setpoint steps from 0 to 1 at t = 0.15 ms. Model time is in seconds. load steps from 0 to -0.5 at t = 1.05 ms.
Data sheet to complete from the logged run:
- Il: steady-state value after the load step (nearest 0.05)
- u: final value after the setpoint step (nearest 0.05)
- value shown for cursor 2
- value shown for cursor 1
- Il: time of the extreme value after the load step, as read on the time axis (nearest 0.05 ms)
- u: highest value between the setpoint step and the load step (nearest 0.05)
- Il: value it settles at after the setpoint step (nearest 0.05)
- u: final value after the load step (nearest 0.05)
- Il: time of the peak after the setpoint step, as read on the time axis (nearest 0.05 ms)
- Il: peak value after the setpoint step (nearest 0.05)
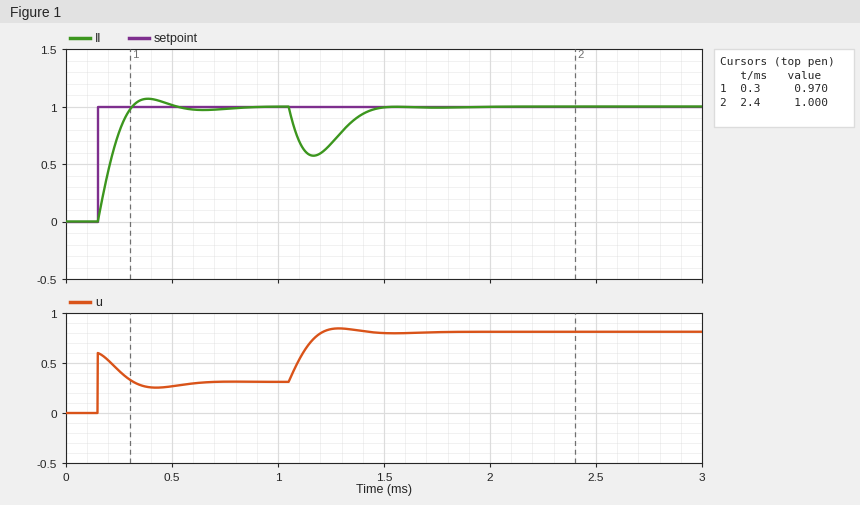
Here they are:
1.00
0.30
1.000
0.970
1.15 ms
0.60
1.00
0.80
0.40 ms
1.05
